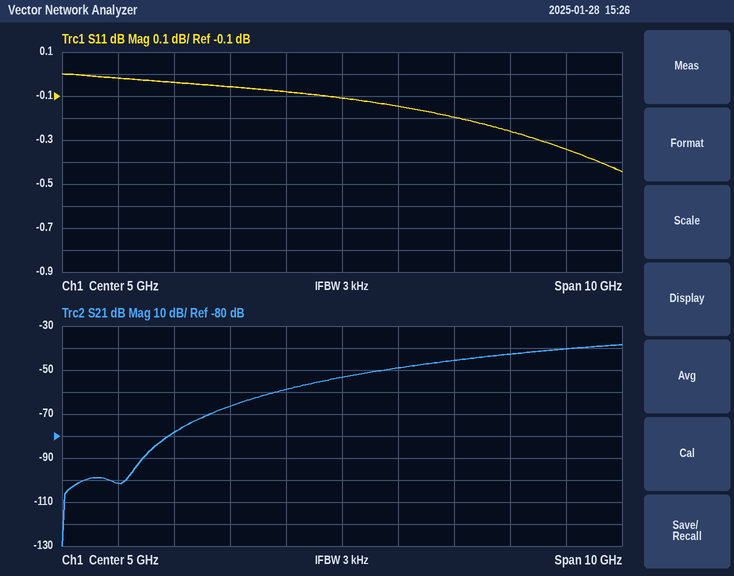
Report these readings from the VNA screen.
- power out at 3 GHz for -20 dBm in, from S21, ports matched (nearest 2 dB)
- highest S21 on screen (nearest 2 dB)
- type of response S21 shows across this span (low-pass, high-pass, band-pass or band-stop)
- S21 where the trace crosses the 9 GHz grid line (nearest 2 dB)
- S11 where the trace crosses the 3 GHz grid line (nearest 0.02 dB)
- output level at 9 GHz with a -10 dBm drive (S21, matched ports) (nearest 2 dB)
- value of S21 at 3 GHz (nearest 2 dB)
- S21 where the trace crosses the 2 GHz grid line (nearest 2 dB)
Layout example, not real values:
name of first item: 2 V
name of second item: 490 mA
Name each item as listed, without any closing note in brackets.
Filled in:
power out at 3 GHz for -20 dBm in, from S21, ports matched: -86 dBm
highest S21 on screen: -38 dB
type of response S21 shows across this span: high-pass
S21 where the trace crosses the 9 GHz grid line: -40 dB
S11 where the trace crosses the 3 GHz grid line: -0.06 dB
output level at 9 GHz with a -10 dBm drive (S21, matched ports): -50 dBm
value of S21 at 3 GHz: -66 dB
S21 where the trace crosses the 2 GHz grid line: -78 dB
